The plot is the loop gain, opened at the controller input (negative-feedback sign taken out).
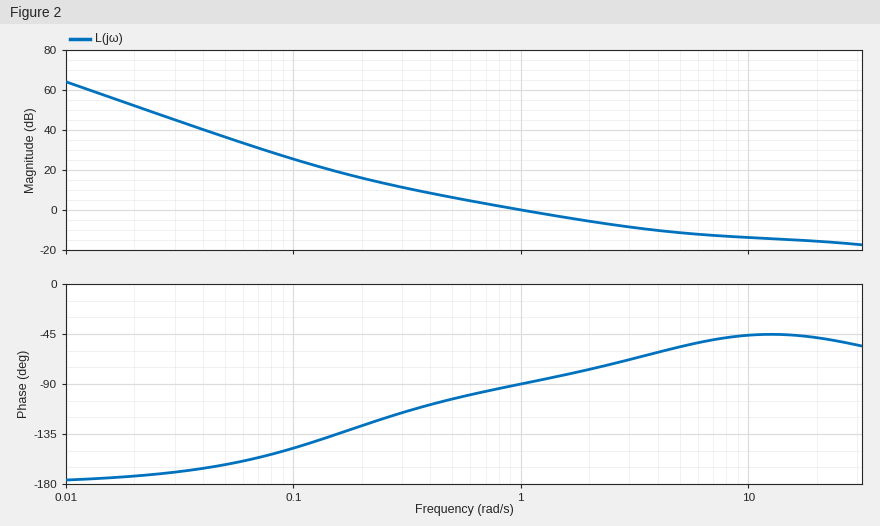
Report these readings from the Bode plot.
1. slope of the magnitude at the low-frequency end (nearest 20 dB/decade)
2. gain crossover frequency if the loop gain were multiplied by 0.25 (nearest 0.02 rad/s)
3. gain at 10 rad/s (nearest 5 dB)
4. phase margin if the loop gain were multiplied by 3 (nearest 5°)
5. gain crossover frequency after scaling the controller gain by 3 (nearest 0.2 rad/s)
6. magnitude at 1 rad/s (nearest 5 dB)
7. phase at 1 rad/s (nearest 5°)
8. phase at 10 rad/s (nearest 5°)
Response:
-40 dB/decade
0.28 rad/s
-15 dB
115°
3.6 rad/s
0 dB
-90°
-45°
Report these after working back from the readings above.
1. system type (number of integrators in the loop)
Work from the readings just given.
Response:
2
